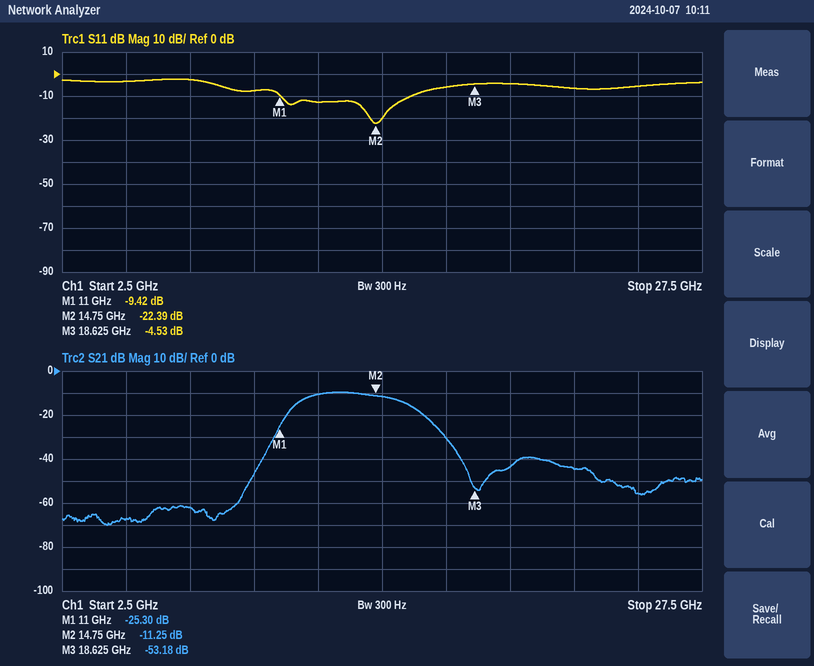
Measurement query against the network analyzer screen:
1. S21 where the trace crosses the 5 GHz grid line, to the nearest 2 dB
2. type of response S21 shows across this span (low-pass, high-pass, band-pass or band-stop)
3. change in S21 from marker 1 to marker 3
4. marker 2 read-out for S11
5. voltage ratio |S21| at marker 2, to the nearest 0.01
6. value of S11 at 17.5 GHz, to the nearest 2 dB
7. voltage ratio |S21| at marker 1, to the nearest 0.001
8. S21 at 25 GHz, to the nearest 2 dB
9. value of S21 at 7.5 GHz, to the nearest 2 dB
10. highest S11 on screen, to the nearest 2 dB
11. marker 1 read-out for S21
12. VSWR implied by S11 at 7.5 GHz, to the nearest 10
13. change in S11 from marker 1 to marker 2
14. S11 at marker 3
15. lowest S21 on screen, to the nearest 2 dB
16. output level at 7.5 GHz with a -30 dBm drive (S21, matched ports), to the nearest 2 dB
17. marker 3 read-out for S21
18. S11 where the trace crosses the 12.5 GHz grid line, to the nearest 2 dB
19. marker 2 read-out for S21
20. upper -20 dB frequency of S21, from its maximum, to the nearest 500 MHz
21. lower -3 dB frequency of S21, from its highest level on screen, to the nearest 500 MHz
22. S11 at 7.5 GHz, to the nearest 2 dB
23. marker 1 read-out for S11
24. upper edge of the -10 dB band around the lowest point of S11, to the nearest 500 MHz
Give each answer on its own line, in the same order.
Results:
-68 dB
band-pass
-27.88 dB
-22.39 dB
0.27
-6 dB
0.054
-56 dB
-62 dB
-2 dB
-25.30 dB
10
-12.97 dB
-4.53 dB
-70 dB
-92 dBm
-53.18 dB
-12 dB
-11.25 dB
17.5 GHz
12.0 GHz
-2 dB
-9.42 dB
16.0 GHz
